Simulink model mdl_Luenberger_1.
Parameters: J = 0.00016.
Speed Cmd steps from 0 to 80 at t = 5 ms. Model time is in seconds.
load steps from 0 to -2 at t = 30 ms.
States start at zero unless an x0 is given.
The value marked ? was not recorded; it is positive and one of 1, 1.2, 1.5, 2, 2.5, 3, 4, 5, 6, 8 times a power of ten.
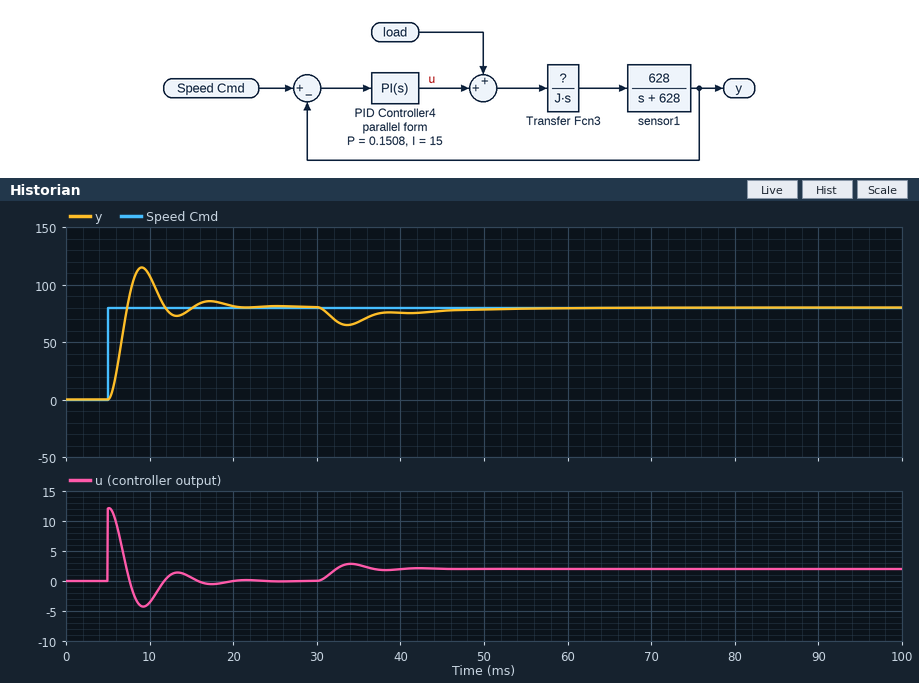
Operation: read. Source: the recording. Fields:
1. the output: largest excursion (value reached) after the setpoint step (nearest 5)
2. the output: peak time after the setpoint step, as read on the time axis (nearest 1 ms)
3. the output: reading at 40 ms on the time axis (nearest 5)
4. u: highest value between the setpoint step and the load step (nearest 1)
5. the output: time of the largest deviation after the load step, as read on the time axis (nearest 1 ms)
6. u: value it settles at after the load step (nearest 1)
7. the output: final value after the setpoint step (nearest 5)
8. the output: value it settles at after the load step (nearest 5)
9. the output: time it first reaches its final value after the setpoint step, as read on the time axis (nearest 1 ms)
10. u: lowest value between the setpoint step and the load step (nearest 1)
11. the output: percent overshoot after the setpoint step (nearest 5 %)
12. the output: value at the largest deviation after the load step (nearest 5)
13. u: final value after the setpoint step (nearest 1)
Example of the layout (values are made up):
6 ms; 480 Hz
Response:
115; 9 ms; 75; 12; 34 ms; 2; 80; 80; 7 ms; -4; 45 %; 65; 0
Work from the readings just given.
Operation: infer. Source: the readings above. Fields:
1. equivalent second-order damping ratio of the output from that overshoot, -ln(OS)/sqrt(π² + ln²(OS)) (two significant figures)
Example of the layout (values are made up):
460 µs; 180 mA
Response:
0.25
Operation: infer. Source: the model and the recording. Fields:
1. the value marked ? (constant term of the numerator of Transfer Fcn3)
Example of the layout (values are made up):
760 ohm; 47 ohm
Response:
1.2
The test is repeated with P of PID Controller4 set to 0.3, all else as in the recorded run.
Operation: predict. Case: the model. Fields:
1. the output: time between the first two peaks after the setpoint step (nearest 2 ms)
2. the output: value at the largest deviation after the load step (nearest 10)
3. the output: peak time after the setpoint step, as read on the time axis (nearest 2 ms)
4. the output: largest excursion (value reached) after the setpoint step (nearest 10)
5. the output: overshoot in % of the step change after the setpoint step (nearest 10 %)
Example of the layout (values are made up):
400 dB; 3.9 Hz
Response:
6 ms; 70; 8 ms; 120; 50 %
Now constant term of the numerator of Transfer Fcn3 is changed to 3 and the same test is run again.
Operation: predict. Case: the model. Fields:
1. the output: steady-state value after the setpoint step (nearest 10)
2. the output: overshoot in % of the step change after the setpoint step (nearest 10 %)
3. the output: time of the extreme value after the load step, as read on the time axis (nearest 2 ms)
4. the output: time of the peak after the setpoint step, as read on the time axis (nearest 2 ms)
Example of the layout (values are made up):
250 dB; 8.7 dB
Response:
80; 60 %; 32 ms; 8 ms
